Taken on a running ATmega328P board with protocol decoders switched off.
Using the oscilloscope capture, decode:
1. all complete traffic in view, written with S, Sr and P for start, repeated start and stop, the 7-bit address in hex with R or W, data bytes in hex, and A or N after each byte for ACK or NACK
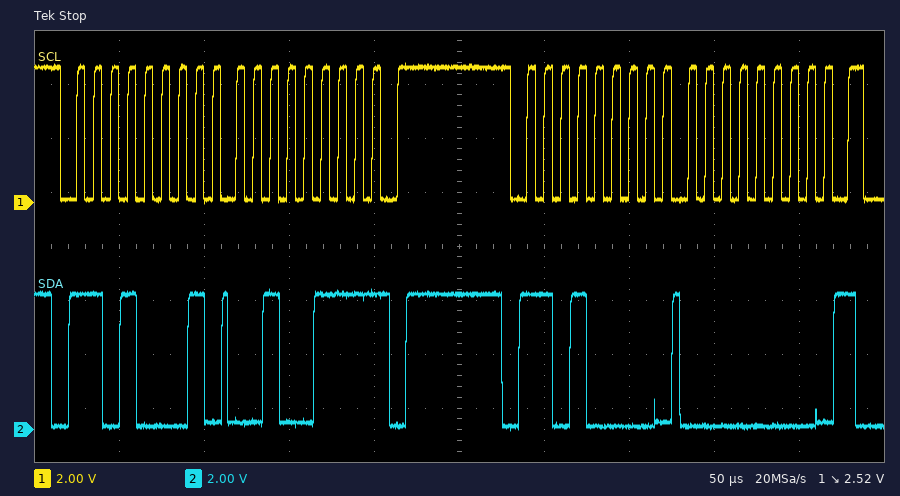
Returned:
S 68R A 27 N P S 68W A 00 A
